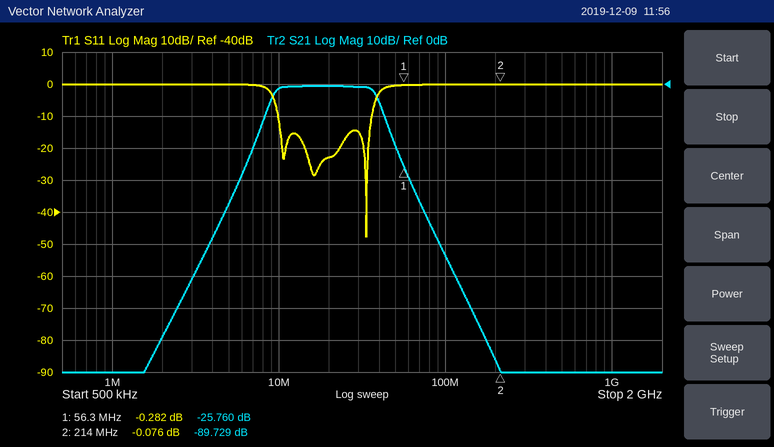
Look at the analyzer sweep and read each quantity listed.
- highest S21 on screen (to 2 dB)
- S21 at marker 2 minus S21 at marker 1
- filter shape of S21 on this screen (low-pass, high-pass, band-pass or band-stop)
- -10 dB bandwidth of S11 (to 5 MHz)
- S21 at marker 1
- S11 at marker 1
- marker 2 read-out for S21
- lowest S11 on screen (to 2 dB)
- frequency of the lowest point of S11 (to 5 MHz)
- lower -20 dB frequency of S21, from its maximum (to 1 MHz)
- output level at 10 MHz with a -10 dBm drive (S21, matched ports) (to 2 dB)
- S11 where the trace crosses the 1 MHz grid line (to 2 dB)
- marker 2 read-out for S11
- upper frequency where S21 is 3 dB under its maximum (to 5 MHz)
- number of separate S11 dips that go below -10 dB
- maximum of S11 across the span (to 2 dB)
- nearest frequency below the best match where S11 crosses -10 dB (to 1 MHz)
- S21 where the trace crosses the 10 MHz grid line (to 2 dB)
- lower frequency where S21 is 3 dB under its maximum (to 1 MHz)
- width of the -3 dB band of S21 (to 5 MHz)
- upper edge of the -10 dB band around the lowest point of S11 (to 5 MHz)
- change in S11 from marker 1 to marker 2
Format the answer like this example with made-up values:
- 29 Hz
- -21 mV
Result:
- 0 dB
- -63.969 dB
- band-pass
- 25 MHz
- -25.760 dB
- -0.282 dB
- -89.729 dB
- -48 dB
- 35 MHz
- 7 MHz
- -12 dBm
- 0 dB
- -0.076 dB
- 40 MHz
- 3
- 0 dB
- 10 MHz
- -2 dB
- 9 MHz
- 30 MHz
- 35 MHz
- 0.206 dB
